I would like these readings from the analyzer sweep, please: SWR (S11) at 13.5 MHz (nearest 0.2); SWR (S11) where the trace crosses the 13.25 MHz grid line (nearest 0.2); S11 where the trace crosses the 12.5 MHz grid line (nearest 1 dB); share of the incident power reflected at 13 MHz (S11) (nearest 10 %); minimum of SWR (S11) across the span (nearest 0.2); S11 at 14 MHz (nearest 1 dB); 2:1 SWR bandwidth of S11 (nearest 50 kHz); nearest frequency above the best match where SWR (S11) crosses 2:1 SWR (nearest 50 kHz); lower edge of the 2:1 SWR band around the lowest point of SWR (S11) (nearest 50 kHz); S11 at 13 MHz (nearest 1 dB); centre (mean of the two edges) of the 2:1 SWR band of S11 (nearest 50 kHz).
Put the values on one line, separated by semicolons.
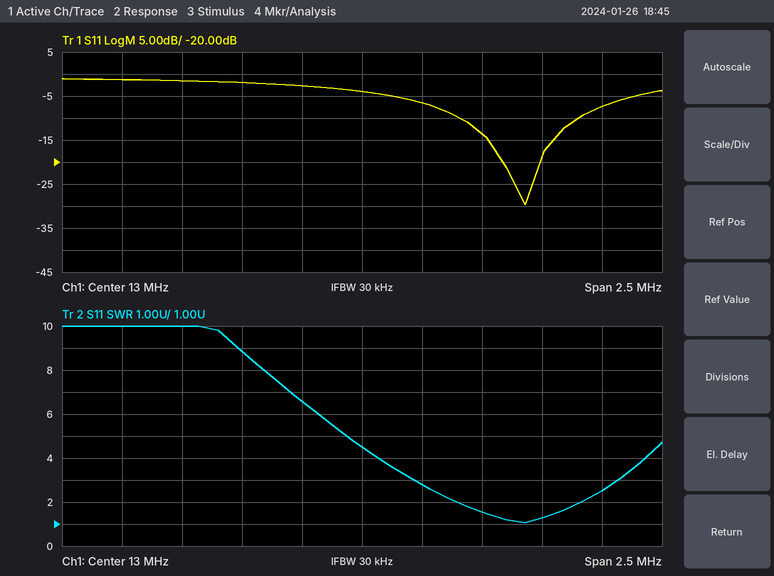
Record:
1.6; 2.8; -2 dB; 40 %; 1.0; -7 dB; 500 kHz; 13.90 MHz; 13.40 MHz; -4 dB; 13.65 MHz
